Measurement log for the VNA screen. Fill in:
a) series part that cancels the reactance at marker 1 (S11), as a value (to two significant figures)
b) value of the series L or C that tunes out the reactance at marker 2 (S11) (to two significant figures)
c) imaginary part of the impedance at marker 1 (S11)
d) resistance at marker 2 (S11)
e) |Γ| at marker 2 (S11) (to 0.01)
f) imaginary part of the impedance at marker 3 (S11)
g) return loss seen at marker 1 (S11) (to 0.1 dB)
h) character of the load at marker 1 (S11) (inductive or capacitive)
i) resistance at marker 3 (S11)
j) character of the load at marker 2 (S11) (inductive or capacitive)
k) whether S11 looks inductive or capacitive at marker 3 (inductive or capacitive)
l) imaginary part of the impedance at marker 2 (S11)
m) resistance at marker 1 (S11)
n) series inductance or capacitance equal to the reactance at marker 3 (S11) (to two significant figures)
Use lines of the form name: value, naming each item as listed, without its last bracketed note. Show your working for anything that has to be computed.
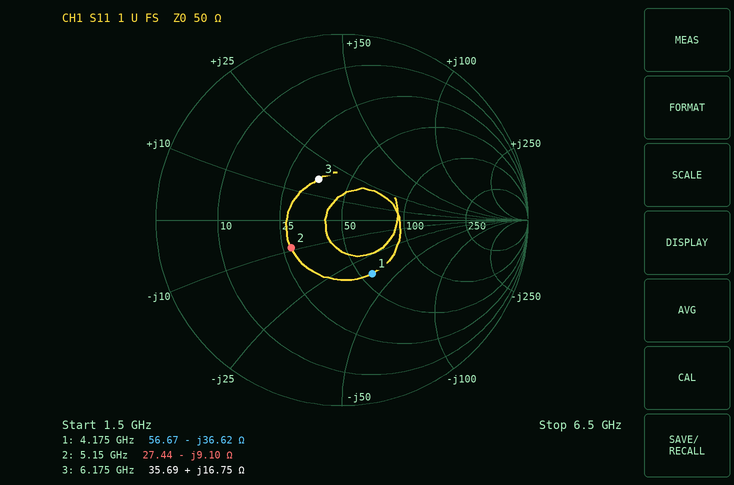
series part that cancels the reactance at marker 1 (S11), as a value: L = 36.62 Ω/(2π × 4.175 GHz) ≈ 1.4 nH
value of the series L or C that tunes out the reactance at marker 2 (S11): L = 9.1 Ω/(2π × 5.15 GHz) ≈ 281 pH, so 280 pH to two significant figures
imaginary part of the impedance at marker 1: -36.62 Ω
resistance at marker 2: 27.44 Ω
|Γ| at marker 2 (S11): 0.31
imaginary part of the impedance at marker 3: +16.75 Ω
return loss seen at marker 1 (S11): 9.6 dB
character of the load at marker 1 (S11): capacitive
resistance at marker 3: 35.69 Ω
character of the load at marker 2 (S11): capacitive
whether S11 looks inductive or capacitive at marker 3: inductive
imaginary part of the impedance at marker 2: -9.10 Ω
resistance at marker 1: 56.67 Ω
series inductance or capacitance equal to the reactance at marker 3 (S11): L = 16.75 Ω/(2π × 6.175 GHz) ≈ 432 pH, so 430 pH to two significant figures
